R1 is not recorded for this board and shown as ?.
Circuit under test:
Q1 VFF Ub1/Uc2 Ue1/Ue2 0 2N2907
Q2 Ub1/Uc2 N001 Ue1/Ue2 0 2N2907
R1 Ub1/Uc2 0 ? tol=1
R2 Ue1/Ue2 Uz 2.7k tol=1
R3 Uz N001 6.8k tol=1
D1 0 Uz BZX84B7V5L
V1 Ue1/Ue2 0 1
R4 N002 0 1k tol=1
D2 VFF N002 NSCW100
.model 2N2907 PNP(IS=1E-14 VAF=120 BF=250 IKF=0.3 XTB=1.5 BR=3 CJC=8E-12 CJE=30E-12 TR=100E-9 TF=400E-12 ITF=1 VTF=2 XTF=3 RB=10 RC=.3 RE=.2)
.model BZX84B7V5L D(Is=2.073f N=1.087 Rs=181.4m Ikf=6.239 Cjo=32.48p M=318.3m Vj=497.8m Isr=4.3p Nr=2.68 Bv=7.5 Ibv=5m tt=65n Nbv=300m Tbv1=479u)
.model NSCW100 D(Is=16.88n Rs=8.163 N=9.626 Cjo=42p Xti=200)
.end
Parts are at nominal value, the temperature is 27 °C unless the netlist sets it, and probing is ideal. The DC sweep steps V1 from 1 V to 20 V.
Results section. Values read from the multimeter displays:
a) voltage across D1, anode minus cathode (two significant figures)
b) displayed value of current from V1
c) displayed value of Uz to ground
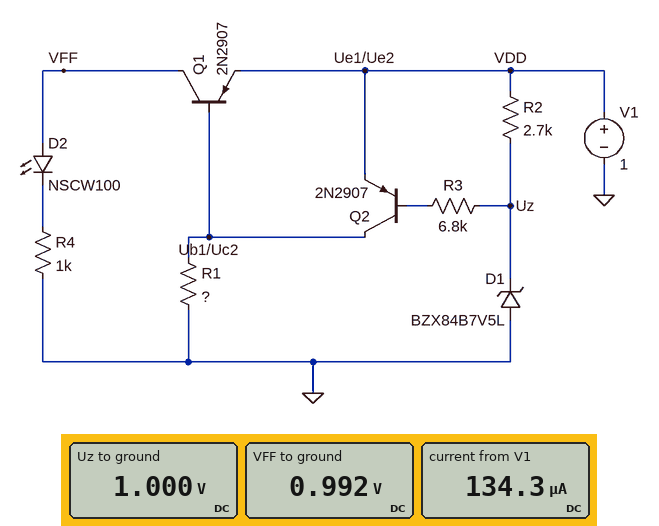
-1.0 V
134.3 µA
1.000 V
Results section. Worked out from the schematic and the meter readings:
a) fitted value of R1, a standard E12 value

2.7 kΩ
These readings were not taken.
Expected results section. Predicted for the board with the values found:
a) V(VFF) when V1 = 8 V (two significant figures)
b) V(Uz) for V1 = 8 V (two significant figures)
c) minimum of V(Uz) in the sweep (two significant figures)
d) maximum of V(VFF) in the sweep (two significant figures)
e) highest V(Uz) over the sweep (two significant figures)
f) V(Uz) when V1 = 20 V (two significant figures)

8.0 V
7.5 V
1.0 V
8.2 V
7.5 V
7.5 V
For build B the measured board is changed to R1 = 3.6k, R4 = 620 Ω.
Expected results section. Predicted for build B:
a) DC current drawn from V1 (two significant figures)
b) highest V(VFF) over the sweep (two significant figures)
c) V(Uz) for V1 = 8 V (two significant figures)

100 µA
8.1 V
7.5 V
